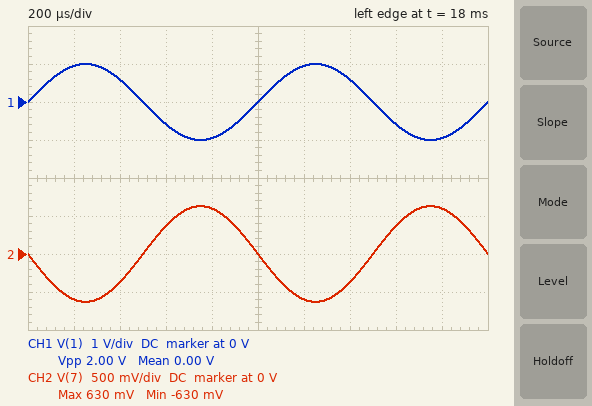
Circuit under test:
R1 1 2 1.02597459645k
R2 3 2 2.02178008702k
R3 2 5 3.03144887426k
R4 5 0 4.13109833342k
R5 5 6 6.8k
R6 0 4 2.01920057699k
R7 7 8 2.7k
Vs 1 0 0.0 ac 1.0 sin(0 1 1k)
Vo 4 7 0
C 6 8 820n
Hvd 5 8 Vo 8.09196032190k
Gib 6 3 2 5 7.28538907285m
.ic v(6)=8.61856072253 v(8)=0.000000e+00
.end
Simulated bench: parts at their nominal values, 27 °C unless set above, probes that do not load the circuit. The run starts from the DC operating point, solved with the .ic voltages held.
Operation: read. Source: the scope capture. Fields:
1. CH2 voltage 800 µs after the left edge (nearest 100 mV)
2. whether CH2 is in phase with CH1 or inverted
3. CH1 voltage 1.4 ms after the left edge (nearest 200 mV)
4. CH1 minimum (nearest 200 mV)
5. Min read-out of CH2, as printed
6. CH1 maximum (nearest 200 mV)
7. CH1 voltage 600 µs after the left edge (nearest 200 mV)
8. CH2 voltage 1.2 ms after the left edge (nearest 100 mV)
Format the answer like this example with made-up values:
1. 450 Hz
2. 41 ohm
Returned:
1. 600 mV
2. inverted
3. 600 mV
4. -1.0 V
5. -630 mV
6. 1.0 V
7. -600 mV
8. -600 mV
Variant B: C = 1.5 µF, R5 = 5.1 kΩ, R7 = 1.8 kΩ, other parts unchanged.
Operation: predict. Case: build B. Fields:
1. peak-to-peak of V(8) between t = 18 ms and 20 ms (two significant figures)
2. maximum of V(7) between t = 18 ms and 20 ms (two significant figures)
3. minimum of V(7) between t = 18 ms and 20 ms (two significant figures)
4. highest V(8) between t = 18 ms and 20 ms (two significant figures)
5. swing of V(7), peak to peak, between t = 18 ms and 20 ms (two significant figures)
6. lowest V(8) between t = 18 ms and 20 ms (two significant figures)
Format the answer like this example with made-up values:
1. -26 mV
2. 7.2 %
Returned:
1. 1.8 V
2. 470 mV
3. -470 mV
4. 890 mV
5. 940 mV
6. -890 mV
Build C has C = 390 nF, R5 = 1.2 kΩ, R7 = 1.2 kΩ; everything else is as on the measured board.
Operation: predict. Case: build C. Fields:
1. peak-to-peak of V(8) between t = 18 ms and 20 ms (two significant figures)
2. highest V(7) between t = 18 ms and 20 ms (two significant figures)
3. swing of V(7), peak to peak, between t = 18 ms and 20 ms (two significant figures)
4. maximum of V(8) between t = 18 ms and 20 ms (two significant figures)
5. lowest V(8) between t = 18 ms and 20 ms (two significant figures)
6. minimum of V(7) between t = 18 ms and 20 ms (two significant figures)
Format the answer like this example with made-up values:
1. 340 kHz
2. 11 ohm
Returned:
1. 1.3 V
2. 400 mV
3. 800 mV
4. 640 mV
5. -640 mV
6. -400 mV
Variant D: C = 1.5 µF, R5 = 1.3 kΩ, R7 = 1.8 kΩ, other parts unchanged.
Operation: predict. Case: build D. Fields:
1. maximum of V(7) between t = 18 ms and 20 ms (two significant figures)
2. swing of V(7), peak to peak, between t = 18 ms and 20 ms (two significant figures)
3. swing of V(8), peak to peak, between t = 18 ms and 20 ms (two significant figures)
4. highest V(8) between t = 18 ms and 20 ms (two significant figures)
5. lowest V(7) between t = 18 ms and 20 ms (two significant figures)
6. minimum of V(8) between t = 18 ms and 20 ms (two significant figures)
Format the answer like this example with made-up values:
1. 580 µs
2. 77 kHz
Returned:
1. 470 mV
2. 940 mV
3. 1.8 V
4. 890 mV
5. -470 mV
6. -890 mV
